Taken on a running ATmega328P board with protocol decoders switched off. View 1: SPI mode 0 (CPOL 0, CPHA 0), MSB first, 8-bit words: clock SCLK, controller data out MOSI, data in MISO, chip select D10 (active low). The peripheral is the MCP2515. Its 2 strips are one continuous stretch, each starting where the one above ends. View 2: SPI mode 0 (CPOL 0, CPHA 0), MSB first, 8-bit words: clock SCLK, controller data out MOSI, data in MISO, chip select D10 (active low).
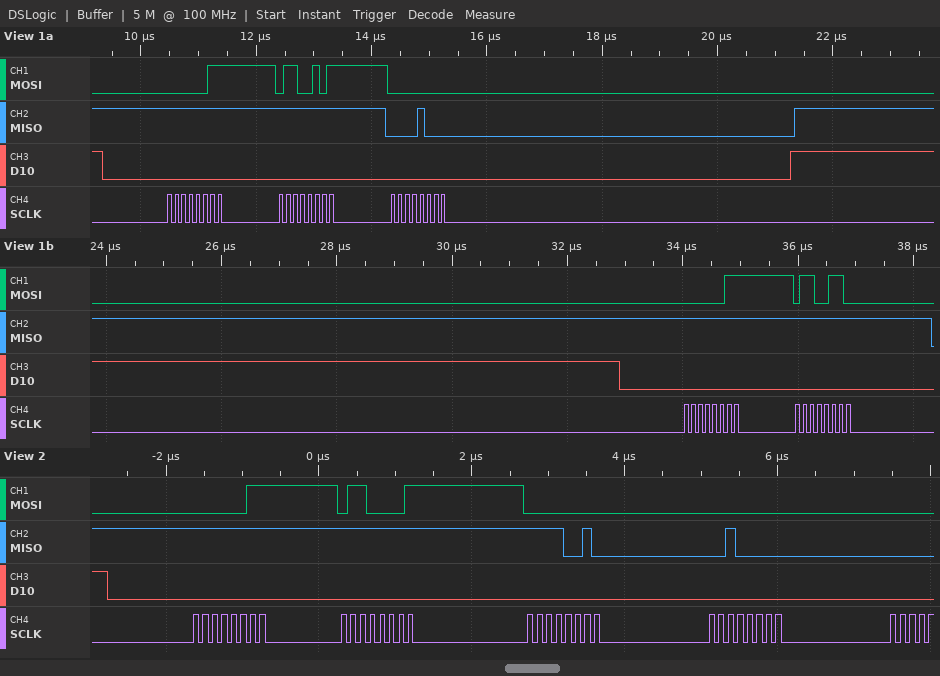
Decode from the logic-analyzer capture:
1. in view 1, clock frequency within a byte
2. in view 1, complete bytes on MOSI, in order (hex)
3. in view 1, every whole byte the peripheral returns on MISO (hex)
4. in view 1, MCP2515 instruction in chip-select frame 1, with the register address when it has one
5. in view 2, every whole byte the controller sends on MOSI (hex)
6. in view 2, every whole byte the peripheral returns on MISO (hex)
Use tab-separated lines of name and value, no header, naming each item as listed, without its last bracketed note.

in view 1, clock frequency within a byte	8 MHz
in view 1, complete bytes on MOSI, in order	03 65 00 03 66
in view 1, every whole byte the peripheral returns on MISO	FF FF 08 FF FF
in view 1, MCP2515 instruction in chip-select frame 1, with the register address when it has one	READ 0x65
in view 2, every whole byte the controller sends on MOSI	0x03 0x61 0x00 0x00
in view 2, every whole byte the peripheral returns on MISO	0xFF 0xFF 0xF2 0x20
